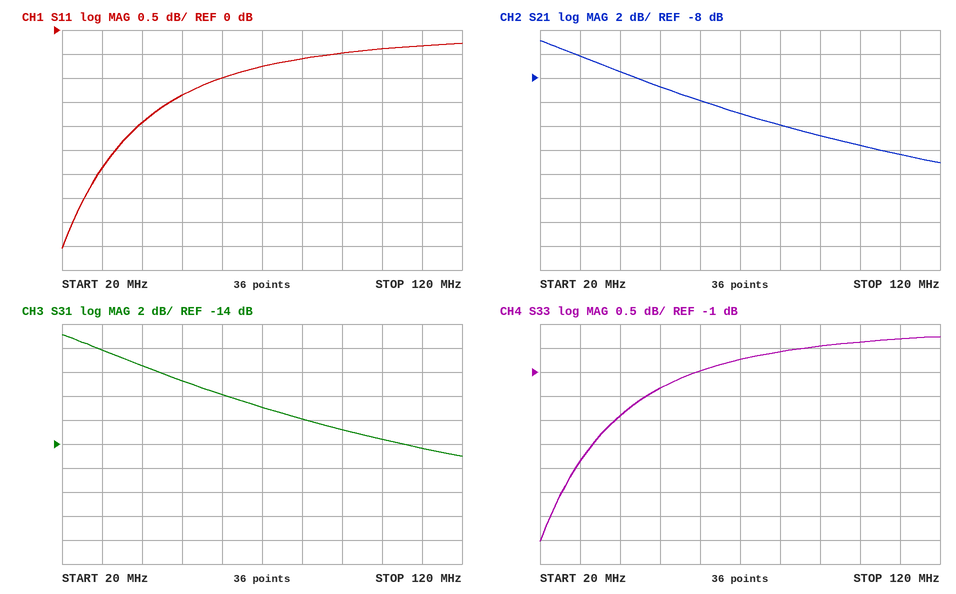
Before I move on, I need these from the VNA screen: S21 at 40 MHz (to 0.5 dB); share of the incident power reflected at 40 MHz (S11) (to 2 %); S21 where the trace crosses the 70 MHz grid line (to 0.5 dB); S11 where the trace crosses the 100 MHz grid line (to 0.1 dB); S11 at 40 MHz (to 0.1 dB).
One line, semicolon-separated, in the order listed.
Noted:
-7.5 dB; 64 %; -11.0 dB; -0.4 dB; -1.9 dB
